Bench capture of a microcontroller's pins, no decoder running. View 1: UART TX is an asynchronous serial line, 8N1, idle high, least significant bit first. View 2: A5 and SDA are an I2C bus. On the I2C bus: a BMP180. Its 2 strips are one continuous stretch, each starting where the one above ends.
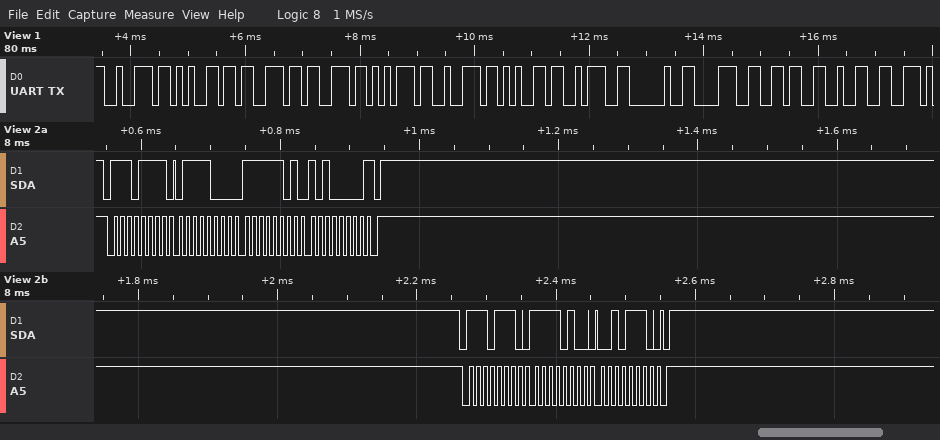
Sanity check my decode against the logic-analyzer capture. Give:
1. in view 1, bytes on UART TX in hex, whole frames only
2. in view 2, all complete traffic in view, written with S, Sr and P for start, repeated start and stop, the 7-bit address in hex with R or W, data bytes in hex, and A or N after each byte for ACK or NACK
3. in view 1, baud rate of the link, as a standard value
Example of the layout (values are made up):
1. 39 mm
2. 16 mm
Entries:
1. 72 65 73 73 75 72 65 3A 20 38 36 32
2. S 77R A 78 A FD A A0 N P S 77W A F4 A 2E A P
3. 9600 baud
